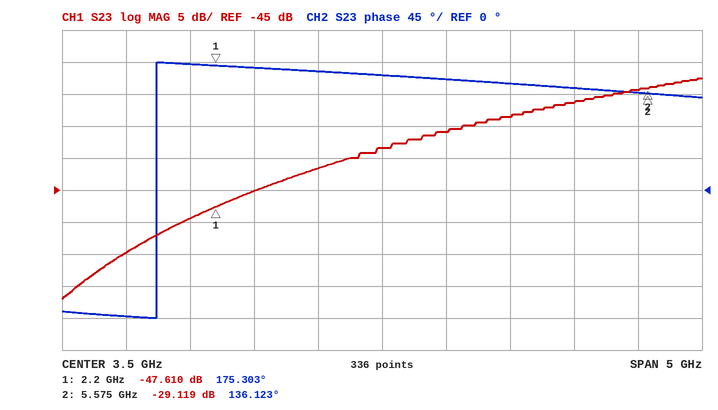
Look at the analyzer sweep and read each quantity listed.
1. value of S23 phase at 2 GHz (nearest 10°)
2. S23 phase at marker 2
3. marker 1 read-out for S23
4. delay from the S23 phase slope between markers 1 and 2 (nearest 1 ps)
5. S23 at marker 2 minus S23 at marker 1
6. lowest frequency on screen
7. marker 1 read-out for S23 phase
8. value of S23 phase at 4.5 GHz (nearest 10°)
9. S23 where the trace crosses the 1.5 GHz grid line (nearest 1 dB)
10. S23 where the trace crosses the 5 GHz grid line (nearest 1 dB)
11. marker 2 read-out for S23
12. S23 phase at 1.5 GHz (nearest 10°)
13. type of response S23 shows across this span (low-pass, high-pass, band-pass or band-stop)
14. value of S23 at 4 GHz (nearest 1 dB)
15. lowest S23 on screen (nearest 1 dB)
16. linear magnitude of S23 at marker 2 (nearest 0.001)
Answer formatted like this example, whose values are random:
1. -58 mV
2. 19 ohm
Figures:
1. 180°
2. 136.123°
3. -47.610 dB
4. 32 ps
5. 18.491 dB
6. 1 GHz
7. 175.303°
8. 150°
9. -55 dB
10. -31 dB
11. -29.119 dB
12. -180°
13. high-pass
14. -36 dB
15. -62 dB
16. 0.035
